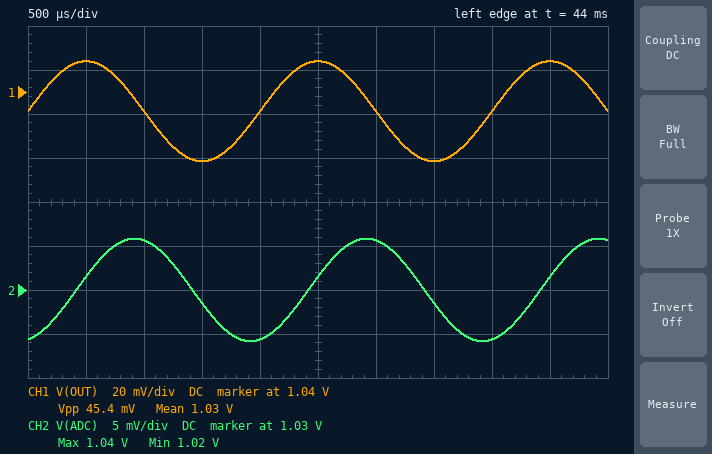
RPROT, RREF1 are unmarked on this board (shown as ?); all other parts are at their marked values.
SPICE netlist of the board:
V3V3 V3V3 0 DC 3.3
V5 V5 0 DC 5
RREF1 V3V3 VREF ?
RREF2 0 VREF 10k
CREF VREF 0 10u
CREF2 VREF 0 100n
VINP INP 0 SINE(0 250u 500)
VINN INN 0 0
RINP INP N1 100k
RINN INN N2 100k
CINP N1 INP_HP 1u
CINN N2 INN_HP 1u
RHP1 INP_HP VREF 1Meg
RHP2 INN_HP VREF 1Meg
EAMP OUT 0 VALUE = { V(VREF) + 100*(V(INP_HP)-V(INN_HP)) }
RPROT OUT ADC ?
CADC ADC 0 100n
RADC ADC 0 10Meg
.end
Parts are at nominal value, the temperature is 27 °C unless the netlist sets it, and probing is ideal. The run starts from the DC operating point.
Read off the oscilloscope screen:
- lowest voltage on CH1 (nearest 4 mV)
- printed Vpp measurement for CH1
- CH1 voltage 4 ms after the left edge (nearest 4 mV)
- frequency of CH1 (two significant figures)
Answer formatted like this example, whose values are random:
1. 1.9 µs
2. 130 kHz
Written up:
1. 1.008 V
2. 45.4 mV
3. 1.032 V
4. 500 Hz
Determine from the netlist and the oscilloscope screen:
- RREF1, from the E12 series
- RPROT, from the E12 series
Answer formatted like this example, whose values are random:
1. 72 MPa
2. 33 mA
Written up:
1. 22 kΩ
2. 12 kΩ
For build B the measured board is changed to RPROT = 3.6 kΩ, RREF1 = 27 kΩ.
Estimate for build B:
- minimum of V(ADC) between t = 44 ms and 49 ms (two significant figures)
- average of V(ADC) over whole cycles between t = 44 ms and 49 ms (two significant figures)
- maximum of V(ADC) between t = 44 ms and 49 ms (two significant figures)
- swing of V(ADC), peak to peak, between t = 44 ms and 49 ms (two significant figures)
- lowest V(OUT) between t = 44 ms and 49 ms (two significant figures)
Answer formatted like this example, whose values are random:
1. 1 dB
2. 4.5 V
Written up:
1. 880 mV
2. 890 mV
3. 910 mV
4. 30 mV
5. 870 mV
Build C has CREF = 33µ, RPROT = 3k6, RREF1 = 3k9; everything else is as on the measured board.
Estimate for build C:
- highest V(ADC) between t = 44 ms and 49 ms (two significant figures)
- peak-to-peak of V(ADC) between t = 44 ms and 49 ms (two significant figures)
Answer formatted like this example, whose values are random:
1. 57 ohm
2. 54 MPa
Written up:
1. 2.4 V
2. 30 mV
